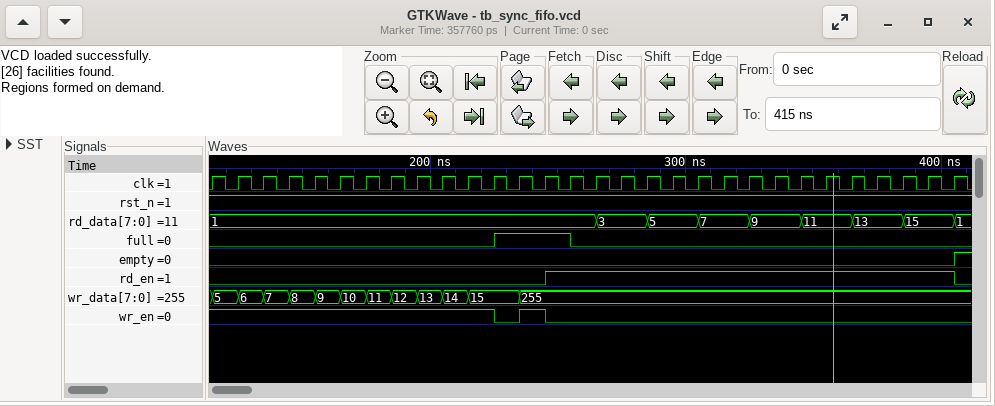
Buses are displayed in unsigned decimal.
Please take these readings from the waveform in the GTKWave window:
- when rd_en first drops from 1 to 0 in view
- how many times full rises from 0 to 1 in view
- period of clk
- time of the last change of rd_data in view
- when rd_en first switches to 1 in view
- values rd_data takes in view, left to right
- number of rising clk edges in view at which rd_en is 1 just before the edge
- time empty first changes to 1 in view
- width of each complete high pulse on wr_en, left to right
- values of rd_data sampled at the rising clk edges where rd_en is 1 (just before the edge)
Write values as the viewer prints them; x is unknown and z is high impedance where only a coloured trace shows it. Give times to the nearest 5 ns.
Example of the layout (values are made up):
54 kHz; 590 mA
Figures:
405 ns; 1; 10 ns; 405 ns; 245 ns; 1, 3, 5, 7, 9, 11, 13, 15, 1; 16; 405 ns; 10 ns; 1, 1, 3, 3, 5, 5, 7, 7, 9, 9, 11, 11, 13, 13, 15, 15
